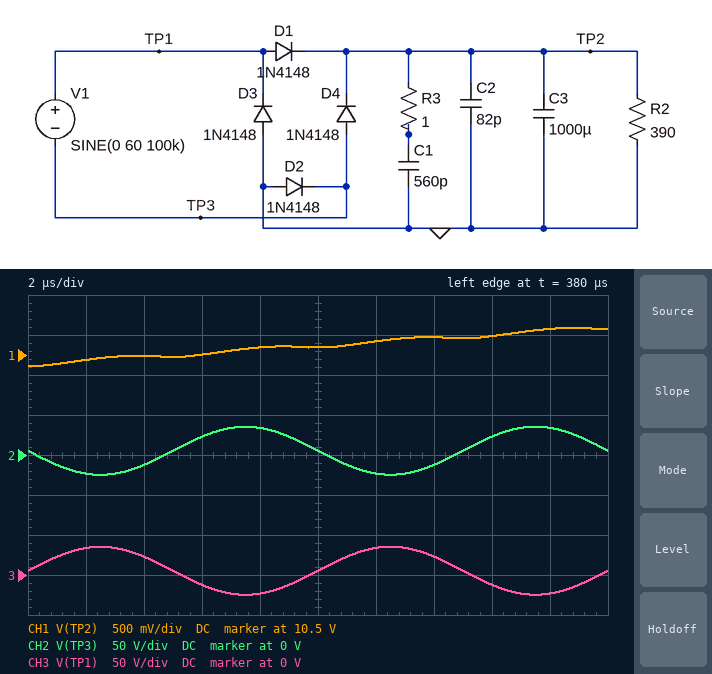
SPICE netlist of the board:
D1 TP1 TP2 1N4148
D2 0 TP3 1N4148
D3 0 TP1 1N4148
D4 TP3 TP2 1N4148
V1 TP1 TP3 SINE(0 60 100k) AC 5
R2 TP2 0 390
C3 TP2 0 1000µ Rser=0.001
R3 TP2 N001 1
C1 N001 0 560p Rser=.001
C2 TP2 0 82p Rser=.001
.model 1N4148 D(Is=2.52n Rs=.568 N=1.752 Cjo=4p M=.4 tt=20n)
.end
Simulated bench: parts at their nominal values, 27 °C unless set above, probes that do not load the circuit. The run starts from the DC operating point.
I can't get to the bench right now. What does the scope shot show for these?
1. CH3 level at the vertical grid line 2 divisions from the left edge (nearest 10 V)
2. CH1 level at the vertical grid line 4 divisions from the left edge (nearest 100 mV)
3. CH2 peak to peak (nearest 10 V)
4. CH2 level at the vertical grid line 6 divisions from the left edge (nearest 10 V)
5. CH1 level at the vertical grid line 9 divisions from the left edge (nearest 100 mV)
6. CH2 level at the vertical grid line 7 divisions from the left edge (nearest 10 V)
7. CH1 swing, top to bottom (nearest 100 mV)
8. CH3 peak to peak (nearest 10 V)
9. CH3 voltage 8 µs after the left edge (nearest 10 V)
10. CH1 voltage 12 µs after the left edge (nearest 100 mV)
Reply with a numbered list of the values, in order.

1. 20 V
2. 10.6 V
3. 60 V
4. -20 V
5. 10.8 V
6. -10 V
7. 500 mV
8. 60 V
9. -20 V
10. 10.7 V
